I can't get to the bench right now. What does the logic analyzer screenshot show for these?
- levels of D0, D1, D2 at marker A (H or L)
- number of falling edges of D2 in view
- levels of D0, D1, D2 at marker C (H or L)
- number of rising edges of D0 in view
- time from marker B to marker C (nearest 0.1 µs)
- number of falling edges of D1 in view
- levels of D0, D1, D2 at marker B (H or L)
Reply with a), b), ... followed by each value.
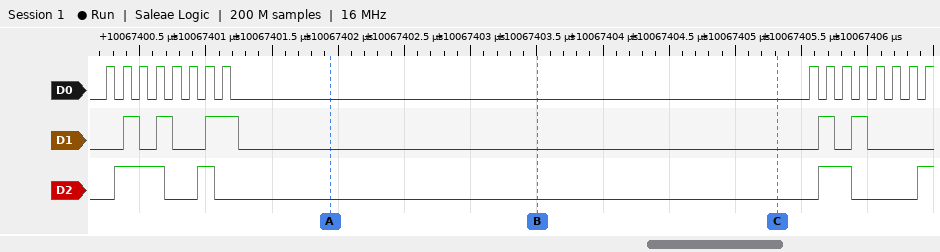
a) D0=L, D1=L, D2=L
b) 3
c) D0=L, D1=L, D2=L
d) 16
e) 1.8 µs
f) 5
g) D0=L, D1=L, D2=L
